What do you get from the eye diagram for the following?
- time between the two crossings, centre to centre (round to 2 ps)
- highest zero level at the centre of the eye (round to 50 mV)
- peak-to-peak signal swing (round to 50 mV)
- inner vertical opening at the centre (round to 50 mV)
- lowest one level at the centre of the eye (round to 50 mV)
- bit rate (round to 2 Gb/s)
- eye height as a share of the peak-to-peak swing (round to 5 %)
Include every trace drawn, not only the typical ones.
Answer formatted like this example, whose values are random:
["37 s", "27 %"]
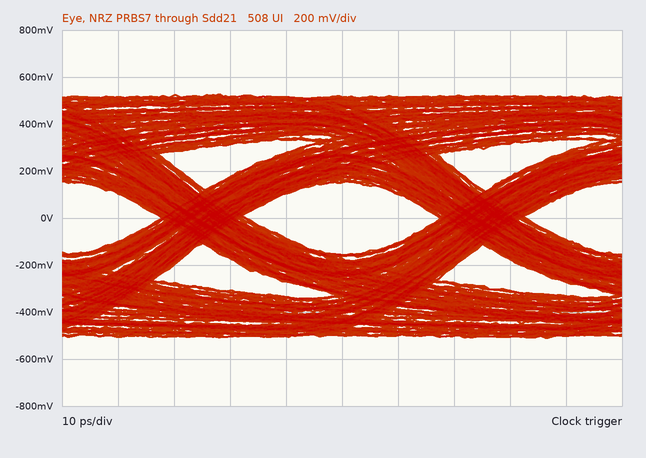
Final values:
["50 ps", "-150 mV", "1.05 V", "300 mV", "150 mV", "20 Gb/s", "30 %"]
